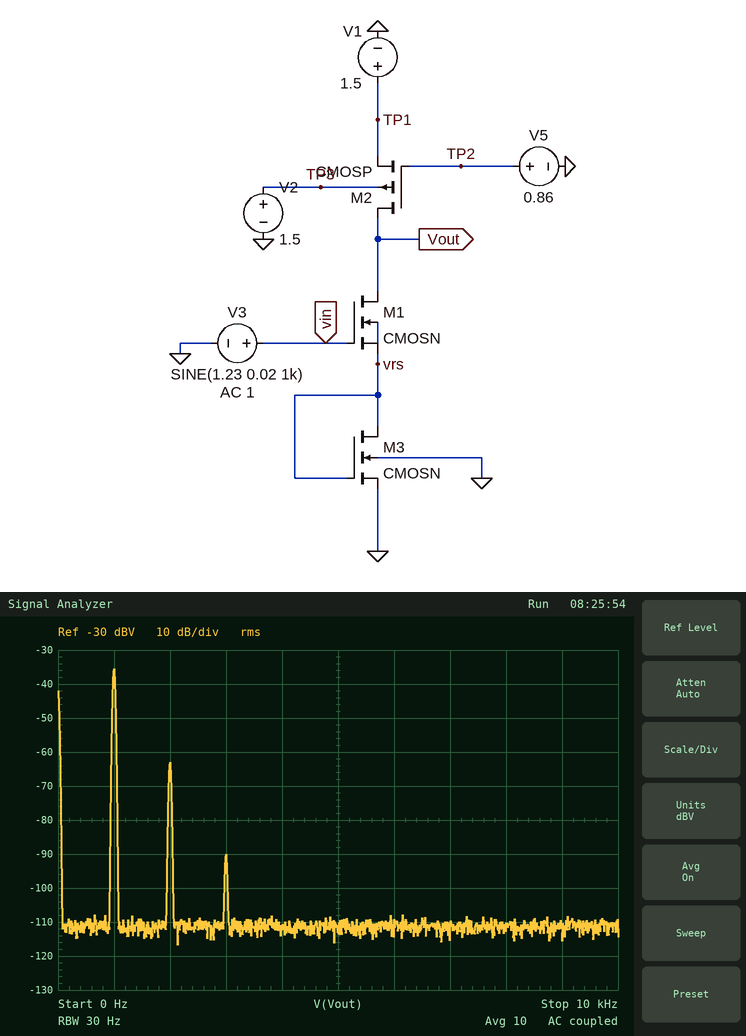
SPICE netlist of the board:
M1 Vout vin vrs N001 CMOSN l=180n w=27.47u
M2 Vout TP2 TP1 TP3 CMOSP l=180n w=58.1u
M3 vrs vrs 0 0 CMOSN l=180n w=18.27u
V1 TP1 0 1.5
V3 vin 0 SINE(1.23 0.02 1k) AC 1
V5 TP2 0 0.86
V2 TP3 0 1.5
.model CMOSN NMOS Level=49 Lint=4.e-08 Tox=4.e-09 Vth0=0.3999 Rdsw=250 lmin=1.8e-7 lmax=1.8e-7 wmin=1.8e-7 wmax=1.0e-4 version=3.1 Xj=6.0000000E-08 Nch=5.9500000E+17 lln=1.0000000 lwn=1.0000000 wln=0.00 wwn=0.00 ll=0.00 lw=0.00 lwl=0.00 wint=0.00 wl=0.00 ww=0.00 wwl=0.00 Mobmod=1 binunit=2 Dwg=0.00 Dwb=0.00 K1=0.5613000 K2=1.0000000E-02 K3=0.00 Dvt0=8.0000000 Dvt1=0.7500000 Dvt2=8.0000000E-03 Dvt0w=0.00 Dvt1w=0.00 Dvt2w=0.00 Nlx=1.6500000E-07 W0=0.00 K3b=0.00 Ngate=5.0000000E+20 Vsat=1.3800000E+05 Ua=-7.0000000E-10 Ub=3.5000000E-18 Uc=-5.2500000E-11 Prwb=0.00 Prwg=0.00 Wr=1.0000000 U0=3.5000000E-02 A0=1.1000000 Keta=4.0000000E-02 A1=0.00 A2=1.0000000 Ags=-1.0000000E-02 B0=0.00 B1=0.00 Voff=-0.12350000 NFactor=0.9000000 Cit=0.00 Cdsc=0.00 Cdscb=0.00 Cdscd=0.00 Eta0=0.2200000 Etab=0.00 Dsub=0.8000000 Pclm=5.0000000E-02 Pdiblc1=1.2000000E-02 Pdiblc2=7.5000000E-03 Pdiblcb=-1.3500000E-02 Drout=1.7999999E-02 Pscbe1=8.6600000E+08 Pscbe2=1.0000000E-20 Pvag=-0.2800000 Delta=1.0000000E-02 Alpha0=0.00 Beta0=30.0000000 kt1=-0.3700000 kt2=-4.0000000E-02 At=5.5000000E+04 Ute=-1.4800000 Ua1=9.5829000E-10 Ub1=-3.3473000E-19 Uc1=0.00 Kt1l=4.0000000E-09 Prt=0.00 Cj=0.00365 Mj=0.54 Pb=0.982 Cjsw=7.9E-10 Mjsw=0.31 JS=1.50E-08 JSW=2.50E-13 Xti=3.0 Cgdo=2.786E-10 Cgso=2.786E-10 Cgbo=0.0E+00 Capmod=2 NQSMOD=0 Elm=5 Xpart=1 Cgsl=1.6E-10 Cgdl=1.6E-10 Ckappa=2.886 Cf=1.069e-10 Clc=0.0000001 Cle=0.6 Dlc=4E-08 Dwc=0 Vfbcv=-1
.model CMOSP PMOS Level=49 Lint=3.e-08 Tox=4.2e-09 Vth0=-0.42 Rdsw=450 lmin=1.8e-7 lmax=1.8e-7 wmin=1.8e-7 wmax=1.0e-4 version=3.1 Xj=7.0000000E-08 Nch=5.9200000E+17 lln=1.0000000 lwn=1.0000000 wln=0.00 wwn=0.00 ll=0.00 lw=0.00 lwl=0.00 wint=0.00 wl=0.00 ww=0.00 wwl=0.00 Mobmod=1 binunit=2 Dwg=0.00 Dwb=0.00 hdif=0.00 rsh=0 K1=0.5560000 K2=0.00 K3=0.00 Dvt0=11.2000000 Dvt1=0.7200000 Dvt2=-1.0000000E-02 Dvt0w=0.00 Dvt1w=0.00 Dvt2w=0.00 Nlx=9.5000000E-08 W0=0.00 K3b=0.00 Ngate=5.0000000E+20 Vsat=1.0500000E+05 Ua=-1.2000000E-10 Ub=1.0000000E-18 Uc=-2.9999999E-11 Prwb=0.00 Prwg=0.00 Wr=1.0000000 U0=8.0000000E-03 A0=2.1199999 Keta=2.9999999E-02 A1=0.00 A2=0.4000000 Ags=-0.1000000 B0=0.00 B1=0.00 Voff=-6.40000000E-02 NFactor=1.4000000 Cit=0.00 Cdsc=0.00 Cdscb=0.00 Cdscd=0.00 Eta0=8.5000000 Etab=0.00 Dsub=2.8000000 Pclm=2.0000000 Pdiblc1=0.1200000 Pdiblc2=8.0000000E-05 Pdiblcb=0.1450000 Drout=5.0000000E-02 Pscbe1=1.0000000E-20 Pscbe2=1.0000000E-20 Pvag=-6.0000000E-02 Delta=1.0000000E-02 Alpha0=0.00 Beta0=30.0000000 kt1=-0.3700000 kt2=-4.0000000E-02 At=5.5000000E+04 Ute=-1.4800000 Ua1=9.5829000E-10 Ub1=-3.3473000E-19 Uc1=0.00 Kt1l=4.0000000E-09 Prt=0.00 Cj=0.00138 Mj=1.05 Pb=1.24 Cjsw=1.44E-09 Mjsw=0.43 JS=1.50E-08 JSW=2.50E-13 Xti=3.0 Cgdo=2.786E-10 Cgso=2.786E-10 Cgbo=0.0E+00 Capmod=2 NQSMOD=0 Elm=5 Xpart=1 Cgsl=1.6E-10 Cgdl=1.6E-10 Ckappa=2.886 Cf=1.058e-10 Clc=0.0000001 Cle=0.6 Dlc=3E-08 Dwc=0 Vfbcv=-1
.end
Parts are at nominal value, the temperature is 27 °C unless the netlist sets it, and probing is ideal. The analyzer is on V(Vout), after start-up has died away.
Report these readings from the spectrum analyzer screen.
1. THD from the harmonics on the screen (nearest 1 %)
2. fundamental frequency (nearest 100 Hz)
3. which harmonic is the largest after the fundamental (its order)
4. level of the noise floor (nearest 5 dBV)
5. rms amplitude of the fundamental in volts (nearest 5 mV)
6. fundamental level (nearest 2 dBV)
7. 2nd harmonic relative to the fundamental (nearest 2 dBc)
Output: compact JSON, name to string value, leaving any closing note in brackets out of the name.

{"THD from the harmonics on the screen": "4 %", "fundamental frequency": "1.0 kHz", "which harmonic is the largest after the fundamental": "2", "level of the noise floor": "-110 dBV", "rms amplitude of the fundamental in volts": "15 mV", "fundamental level": "-36 dBV", "2nd harmonic relative to the fundamental": "-28 dBc"}
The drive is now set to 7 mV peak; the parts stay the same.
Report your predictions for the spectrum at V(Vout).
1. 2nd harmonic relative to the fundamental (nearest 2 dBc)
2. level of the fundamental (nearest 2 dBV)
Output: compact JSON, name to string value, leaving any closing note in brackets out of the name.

{"2nd harmonic relative to the fundamental": "-36 dBc", "level of the fundamental": "-44 dBV"}
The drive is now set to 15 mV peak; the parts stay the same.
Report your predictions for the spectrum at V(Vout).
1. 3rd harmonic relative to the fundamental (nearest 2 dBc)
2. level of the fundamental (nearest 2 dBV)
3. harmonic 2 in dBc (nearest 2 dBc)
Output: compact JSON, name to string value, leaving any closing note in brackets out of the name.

{"3rd harmonic relative to the fundamental": "-60 dBc", "level of the fundamental": "-38 dBV", "harmonic 2 in dBc": "-30 dBc"}
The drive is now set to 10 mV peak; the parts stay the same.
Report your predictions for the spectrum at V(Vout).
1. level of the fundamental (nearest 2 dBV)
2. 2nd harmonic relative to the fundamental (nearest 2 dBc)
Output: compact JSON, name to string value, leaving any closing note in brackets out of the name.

{"level of the fundamental": "-42 dBV", "2nd harmonic relative to the fundamental": "-34 dBc"}
